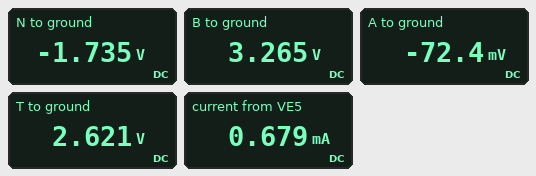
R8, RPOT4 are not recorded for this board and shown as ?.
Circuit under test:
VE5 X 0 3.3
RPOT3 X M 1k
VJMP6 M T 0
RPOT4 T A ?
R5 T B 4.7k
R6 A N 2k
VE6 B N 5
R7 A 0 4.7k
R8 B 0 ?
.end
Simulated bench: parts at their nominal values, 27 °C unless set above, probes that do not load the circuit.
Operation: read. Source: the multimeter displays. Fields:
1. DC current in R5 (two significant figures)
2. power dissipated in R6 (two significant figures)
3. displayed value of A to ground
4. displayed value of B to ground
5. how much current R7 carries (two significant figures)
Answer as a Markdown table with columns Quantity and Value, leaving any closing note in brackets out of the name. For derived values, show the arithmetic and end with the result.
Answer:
| Quantity | Value |
|---|---|
| DC current in R5 | (3.265 V - 2.621 V) / 4.7 kΩ = 140 µA |
| power dissipated in R6 | (-72.4 mV - (-1.735 V))^2 / 2 kΩ = 1.4 mW |
| displayed value of A to ground | -72.4 mV |
| displayed value of B to ground | 3.265 V |
| how much current R7 carries | (0 V - (-72.4 mV)) / 4.7 kΩ = 15 µA |
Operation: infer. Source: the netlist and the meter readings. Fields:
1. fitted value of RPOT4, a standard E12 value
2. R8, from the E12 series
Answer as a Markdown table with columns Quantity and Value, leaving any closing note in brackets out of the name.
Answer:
| Quantity | Value |
|---|---|
| fitted value of RPOT4, a standard E12 value | 3.3 kΩ |
| R8, from the E12 series | 4.7 kΩ |
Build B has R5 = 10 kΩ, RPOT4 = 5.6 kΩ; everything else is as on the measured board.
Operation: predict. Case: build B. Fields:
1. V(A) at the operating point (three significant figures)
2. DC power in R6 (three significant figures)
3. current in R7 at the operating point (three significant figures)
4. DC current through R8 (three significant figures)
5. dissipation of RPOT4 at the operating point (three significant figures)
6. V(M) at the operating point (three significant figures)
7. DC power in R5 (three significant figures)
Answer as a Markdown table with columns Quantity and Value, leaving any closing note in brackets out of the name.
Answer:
| Quantity | Value |
|---|---|
| V(A) at the operating point | -517 mV |
| DC power in R6 | 962 µW |
| current in R7 at the operating point | 110 µA |
| DC current through R8 | 659 µA |
| dissipation of RPOT4 at the operating point | 1.91 mW |
| V(M) at the operating point | 2.75 V |
| DC power in R5 | 11.9 µW |
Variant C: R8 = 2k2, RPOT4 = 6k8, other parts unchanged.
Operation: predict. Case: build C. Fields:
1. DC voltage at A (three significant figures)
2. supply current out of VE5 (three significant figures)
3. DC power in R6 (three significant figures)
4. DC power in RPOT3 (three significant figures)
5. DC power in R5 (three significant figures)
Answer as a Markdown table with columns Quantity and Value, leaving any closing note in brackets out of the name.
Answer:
| Quantity | Value |
|---|---|
| DC voltage at A | -1.25 V |
| supply current out of VE5 | 682 µA |
| DC power in R6 | 1.39 mW |
| DC power in RPOT3 | 465 µW |
| DC power in R5 | 60.6 µW |
